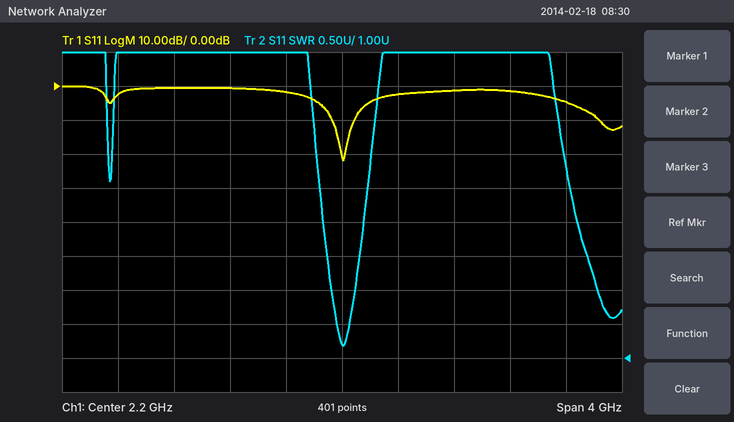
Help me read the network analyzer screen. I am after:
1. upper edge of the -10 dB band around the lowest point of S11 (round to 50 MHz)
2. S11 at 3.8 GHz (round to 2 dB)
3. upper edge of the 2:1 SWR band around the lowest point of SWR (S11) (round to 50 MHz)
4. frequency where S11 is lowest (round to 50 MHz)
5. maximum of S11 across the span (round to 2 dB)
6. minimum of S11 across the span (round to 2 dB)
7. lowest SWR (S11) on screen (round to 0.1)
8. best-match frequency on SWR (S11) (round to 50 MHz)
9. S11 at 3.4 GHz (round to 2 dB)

2.30 GHz
-4 dB
2.30 GHz
2.20 GHz
0 dB
-22 dB
1.2
2.20 GHz
-2 dB
